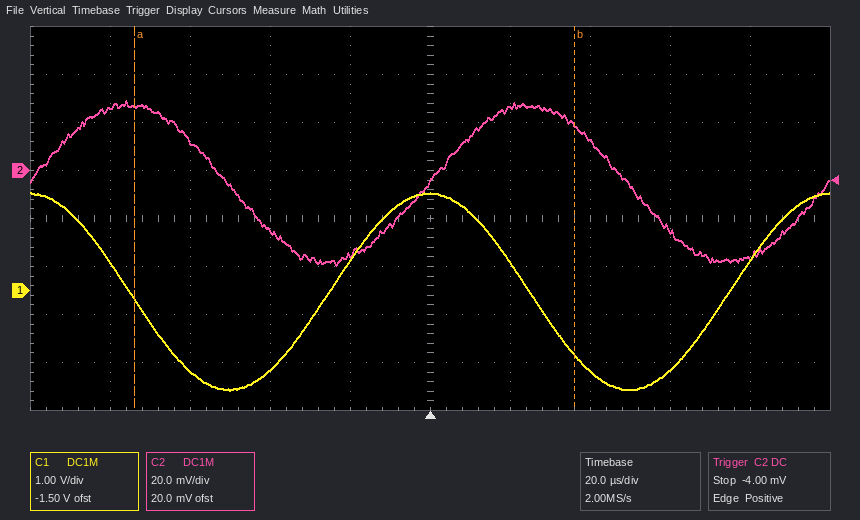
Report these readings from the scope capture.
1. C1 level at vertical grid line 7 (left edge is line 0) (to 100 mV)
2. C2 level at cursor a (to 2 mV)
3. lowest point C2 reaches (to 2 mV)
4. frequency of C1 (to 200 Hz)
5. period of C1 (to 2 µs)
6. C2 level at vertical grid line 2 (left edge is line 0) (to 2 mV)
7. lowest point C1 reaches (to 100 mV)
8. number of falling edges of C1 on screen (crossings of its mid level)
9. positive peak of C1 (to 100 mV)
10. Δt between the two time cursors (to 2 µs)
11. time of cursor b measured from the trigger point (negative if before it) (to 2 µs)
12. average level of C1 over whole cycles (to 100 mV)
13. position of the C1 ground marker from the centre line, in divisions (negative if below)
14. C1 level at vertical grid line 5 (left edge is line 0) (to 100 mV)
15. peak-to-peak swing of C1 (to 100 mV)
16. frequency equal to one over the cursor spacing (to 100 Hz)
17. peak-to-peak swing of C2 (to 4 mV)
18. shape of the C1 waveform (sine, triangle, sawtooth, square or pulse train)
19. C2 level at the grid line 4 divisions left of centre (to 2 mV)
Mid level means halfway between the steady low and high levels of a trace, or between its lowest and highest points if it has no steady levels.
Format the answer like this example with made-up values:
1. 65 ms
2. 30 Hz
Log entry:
1. -1.7 V
2. 26 mV
3. -40 mV
4. 10.0 kHz
5. 100 µs
6. 12 mV
7. -2.1 V
8. 2
9. 2.0 V
10. 110 µs
11. +36 µs
12. 0.0 V
13. -1.5 div
14. 2.0 V
15. 4.1 V
16. 9.1 kHz
17. 68 mV
18. sine
19. 26 mV
